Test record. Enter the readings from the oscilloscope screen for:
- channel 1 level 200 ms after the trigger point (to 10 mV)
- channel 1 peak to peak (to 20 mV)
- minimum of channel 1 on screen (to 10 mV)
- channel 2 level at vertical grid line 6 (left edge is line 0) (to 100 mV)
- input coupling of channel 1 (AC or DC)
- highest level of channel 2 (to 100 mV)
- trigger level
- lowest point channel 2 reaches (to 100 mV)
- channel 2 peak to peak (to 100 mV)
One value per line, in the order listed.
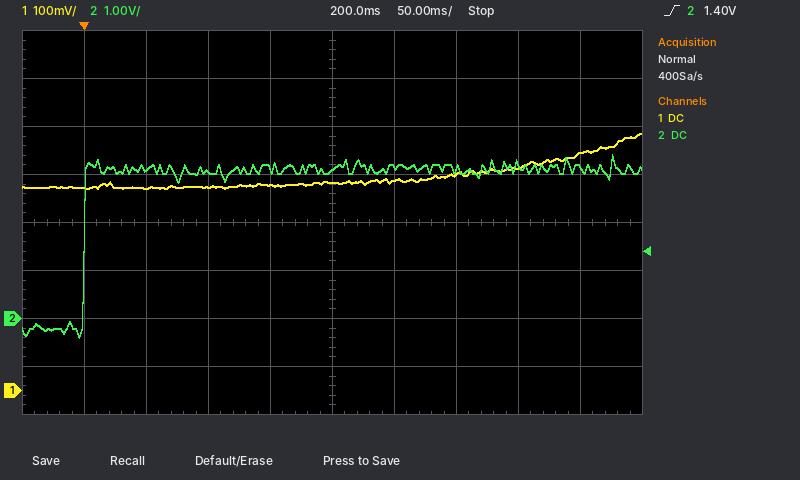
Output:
430 mV
120 mV
420 mV
3.2 V
DC
3.4 V
1.40 V
-400 mV
3.8 V
